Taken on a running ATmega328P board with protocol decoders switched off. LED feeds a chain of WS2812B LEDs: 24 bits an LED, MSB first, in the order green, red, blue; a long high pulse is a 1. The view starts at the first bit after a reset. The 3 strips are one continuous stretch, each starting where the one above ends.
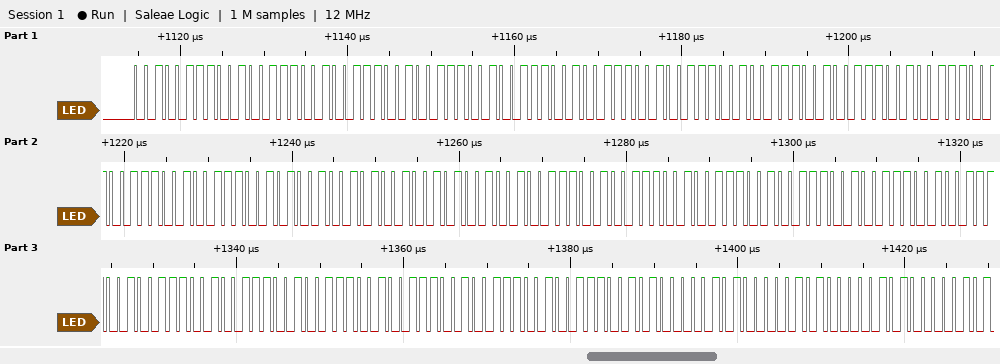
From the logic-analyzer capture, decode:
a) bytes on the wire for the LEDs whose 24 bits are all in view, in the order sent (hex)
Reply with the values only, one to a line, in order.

27 27 27 27 27 27 27 27 27 27 27 27 29 29 29 27 27 27 27 27 27 27 27 27 27 27 27 28 28 28
